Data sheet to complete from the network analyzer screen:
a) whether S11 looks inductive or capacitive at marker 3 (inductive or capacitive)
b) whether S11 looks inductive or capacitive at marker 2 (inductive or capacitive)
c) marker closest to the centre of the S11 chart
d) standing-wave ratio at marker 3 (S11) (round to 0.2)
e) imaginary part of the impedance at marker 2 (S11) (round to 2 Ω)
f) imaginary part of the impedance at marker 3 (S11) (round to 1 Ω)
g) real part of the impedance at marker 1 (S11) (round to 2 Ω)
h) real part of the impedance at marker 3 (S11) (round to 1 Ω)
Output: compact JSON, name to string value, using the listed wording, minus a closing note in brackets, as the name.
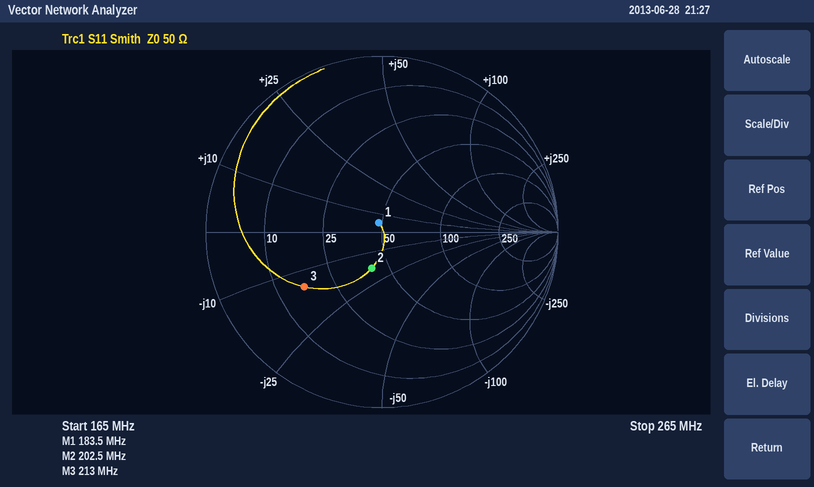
{"whether S11 looks inductive or capacitive at marker 3": "capacitive", "whether S11 looks inductive or capacitive at marker 2": "capacitive", "marker closest to the centre of the S11 chart": "marker 1", "standing-wave ratio at marker 3 (S11)": "3.4", "imaginary part of the impedance at marker 2 (S11)": "-18 Ω", "imaginary part of the impedance at marker 3 (S11)": "-14 Ω", "real part of the impedance at marker 1 (S11)": "48 Ω", "real part of the impedance at marker 3 (S11)": "16 Ω"}
